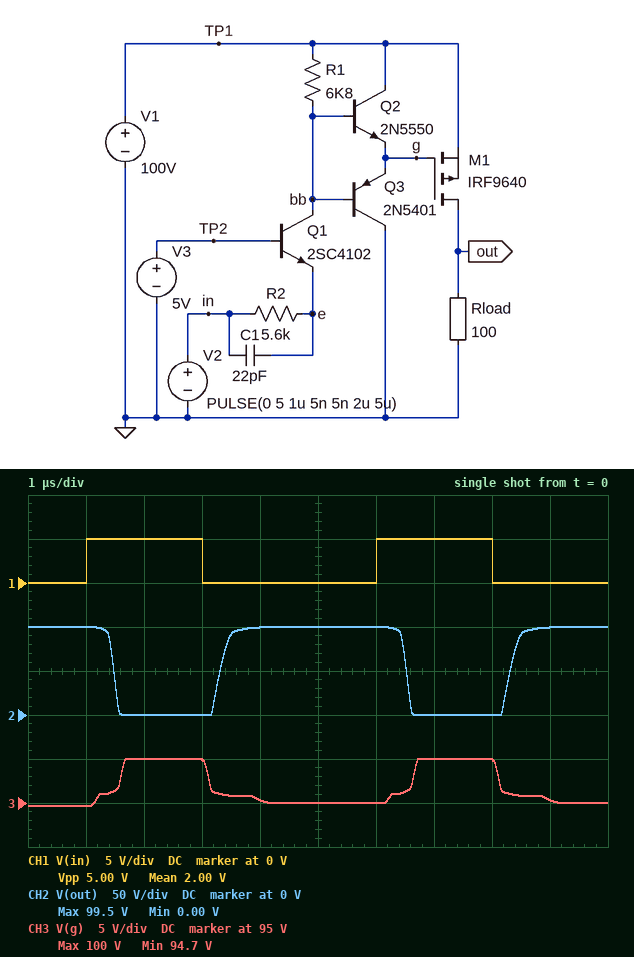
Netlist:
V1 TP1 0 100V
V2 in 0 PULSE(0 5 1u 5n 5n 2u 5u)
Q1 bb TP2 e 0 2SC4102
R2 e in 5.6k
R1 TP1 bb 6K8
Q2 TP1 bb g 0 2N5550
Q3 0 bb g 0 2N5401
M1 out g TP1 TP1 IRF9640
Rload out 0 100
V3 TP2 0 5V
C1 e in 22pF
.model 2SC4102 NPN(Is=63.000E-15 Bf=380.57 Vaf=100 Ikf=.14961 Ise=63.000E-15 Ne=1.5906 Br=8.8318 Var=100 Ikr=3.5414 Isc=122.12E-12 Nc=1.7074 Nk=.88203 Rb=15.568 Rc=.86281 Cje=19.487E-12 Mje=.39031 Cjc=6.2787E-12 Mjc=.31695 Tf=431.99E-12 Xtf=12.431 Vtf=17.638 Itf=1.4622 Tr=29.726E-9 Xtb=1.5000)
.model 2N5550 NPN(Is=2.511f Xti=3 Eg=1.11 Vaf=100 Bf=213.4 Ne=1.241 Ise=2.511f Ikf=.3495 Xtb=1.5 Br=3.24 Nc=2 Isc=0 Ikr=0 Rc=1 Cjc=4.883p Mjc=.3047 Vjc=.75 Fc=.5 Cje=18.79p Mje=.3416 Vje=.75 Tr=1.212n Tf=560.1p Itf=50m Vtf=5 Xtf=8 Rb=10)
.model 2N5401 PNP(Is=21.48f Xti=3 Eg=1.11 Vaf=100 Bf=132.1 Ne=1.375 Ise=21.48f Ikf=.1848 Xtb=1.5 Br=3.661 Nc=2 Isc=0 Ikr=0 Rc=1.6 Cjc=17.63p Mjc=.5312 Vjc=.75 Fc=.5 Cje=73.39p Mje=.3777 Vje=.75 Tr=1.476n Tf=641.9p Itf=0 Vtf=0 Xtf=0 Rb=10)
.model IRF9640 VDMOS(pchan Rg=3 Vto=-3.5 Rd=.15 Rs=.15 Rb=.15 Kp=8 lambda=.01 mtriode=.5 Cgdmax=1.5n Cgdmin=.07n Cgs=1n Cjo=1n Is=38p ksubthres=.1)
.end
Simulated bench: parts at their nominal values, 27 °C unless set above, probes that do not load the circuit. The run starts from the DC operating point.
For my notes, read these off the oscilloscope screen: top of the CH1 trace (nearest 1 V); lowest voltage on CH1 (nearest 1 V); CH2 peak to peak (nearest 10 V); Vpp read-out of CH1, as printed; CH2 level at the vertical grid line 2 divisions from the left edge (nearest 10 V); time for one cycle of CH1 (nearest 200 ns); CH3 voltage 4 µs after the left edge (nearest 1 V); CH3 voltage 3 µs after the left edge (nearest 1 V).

5 V
0 V
100 V
5.00 V
0 V
5.0 µs
95 V
100 V
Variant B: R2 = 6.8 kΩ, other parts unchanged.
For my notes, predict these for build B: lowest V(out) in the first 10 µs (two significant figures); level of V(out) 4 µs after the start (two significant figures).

-180 mV
48 V
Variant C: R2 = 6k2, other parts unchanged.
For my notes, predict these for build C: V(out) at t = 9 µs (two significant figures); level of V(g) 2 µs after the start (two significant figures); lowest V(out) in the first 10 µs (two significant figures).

92 V
100 V
-200 mV
